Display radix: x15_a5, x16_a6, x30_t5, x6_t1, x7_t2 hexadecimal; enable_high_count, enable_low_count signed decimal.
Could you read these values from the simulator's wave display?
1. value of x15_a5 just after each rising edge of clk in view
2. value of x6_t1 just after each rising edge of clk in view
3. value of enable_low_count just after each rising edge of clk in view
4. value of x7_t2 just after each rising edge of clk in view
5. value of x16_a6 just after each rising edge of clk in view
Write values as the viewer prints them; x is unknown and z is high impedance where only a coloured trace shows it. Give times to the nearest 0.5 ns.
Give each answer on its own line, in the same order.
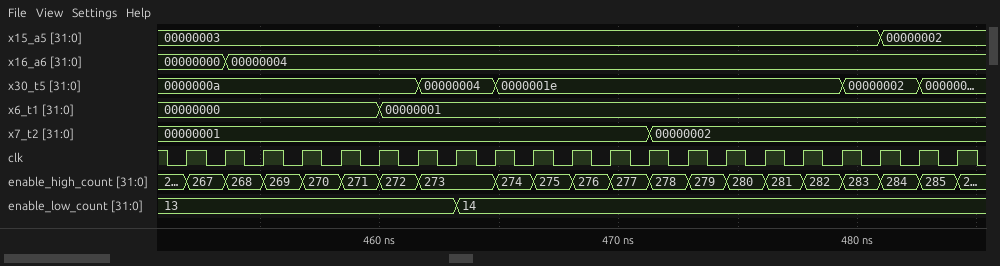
00000003, 00000003, 00000003, 00000003, 00000003, 00000003, 00000003, 00000003, 00000003, 00000003, 00000003, 00000003, 00000003, 00000003, 00000003, 00000003, 00000003, 00000003, 00000002, 00000002, 00000002
00000000, 00000000, 00000000, 00000000, 00000000, 00000001, 00000001, 00000001, 00000001, 00000001, 00000001, 00000001, 00000001, 00000001, 00000001, 00000001, 00000001, 00000001, 00000001, 00000001, 00000001
13, 13, 13, 13, 13, 13, 13, 14, 14, 14, 14, 14, 14, 14, 14, 14, 14, 14, 14, 14, 14
00000001, 00000001, 00000001, 00000001, 00000001, 00000001, 00000001, 00000001, 00000001, 00000001, 00000001, 00000001, 00000002, 00000002, 00000002, 00000002, 00000002, 00000002, 00000002, 00000002, 00000002
00000000, 00000004, 00000004, 00000004, 00000004, 00000004, 00000004, 00000004, 00000004, 00000004, 00000004, 00000004, 00000004, 00000004, 00000004, 00000004, 00000004, 00000004, 00000004, 00000004, 00000004
